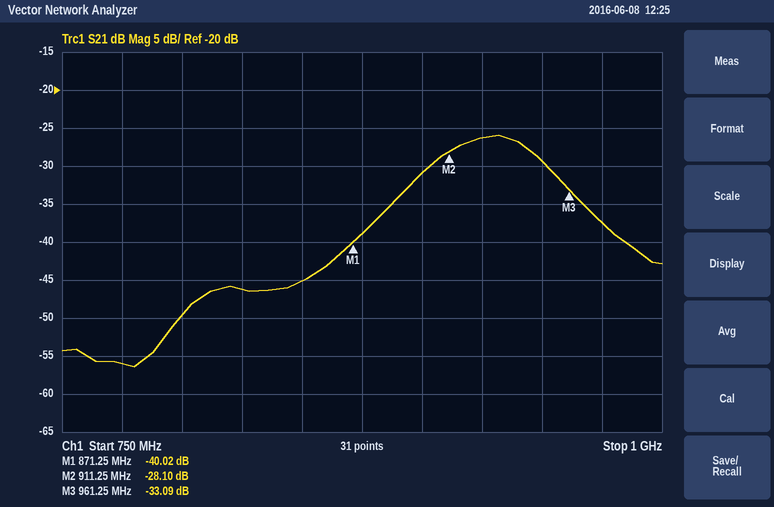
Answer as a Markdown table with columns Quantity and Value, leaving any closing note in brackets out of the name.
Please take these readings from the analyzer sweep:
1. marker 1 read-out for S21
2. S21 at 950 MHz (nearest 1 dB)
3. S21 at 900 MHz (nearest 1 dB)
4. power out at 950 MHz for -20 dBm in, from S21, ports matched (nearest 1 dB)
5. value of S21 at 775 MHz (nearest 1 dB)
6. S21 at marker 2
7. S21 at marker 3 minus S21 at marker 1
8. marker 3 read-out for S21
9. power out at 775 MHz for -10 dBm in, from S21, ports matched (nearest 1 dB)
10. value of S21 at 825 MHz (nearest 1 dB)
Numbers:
| Quantity | Value |
|---|---|
| marker 1 read-out for S21 | -40.02 dB |
| S21 at 950 MHz | -29 dB |
| S21 at 900 MHz | -31 dB |
| power out at 950 MHz for -20 dBm in, from S21, ports matched | -49 dBm |
| value of S21 at 775 MHz | -56 dB |
| S21 at marker 2 | -28.10 dB |
| S21 at marker 3 minus S21 at marker 1 | 6.93 dB |
| marker 3 read-out for S21 | -33.09 dB |
| power out at 775 MHz for -10 dBm in, from S21, ports matched | -66 dBm |
| value of S21 at 825 MHz | -46 dB |
